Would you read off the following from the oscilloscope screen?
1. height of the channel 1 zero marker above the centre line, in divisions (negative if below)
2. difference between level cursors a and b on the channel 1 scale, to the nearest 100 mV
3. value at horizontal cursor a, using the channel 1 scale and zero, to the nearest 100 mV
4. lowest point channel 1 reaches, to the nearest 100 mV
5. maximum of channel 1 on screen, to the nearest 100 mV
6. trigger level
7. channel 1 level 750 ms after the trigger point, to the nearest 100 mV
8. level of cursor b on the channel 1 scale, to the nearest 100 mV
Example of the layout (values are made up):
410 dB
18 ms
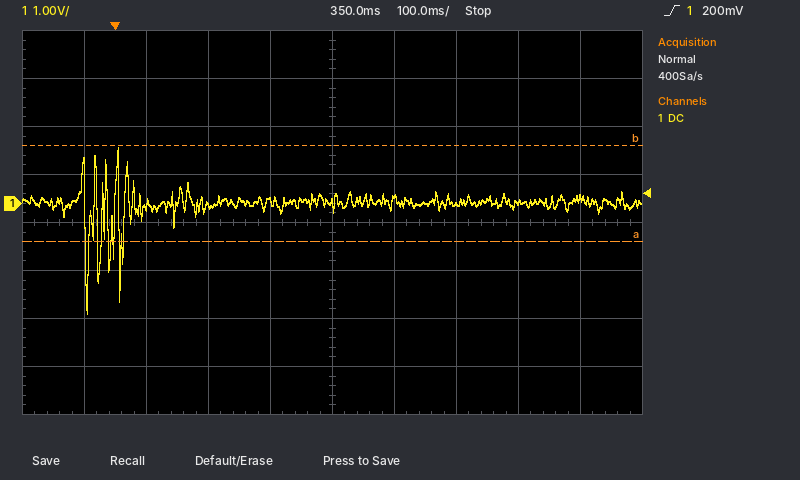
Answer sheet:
+0.4 div
2.0 V
-800 mV
-2.3 V
1.2 V
200 mV
100 mV
1.2 V
